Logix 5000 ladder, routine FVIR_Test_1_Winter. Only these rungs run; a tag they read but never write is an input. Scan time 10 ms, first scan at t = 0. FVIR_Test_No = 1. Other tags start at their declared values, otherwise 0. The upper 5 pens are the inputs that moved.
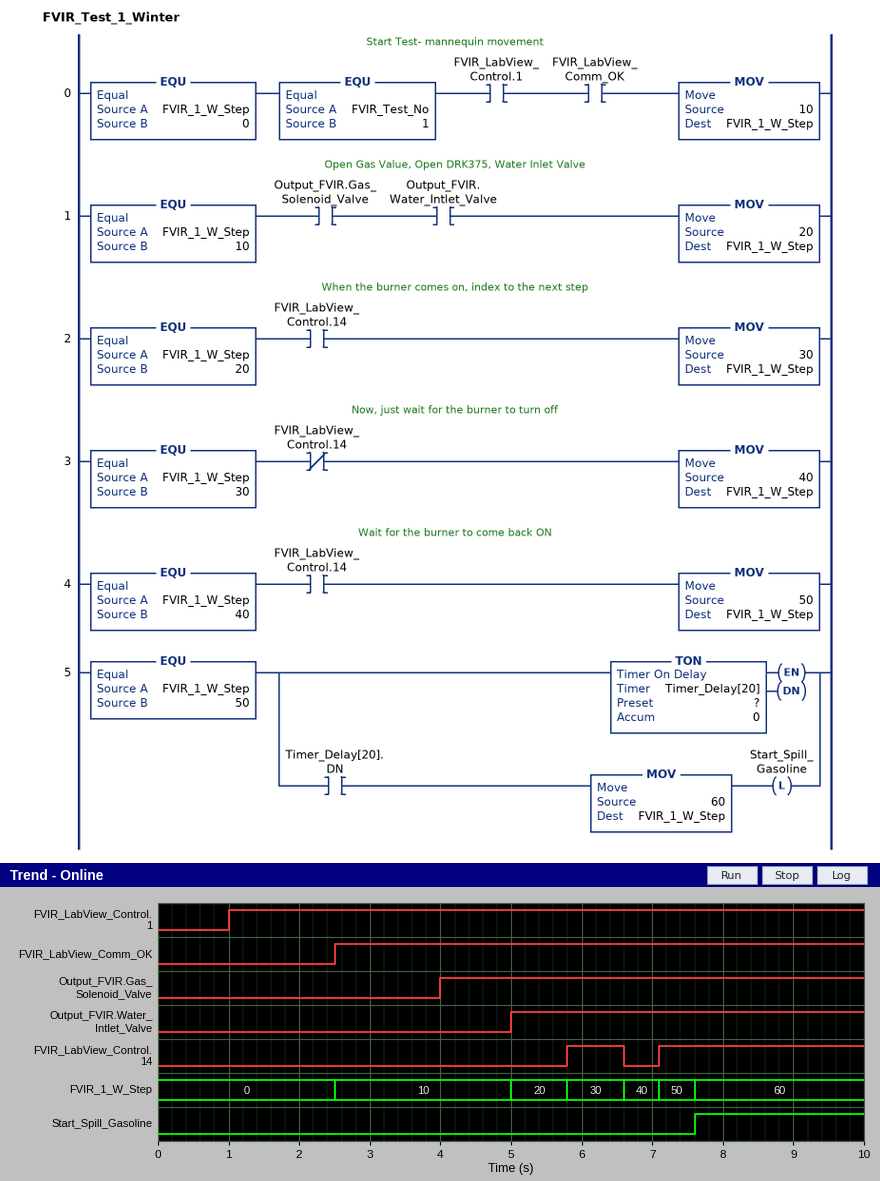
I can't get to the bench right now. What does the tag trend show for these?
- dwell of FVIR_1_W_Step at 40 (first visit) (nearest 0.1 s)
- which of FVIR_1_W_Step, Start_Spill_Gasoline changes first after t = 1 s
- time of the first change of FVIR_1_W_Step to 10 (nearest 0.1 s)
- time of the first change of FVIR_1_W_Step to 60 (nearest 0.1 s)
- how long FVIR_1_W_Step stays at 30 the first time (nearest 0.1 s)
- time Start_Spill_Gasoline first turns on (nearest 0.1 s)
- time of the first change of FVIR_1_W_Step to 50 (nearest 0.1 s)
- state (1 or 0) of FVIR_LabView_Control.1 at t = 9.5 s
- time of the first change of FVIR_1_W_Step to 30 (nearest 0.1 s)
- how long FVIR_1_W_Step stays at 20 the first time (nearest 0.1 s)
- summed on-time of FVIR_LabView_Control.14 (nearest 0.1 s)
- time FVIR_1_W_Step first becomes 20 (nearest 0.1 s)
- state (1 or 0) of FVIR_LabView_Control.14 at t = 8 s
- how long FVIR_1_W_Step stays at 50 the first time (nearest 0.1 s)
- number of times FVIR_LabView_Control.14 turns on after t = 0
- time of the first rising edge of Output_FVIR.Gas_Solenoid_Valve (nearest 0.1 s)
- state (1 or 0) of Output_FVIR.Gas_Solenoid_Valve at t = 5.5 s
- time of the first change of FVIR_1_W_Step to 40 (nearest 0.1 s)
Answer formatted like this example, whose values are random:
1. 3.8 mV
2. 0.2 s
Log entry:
1. 0.5 s
2. FVIR_1_W_Step
3. 2.5 s
4. 7.6 s
5. 0.8 s
6. 7.6 s
7. 7.1 s
8. 1
9. 5.8 s
10. 0.8 s
11. 3.7 s
12. 5.0 s
13. 1
14. 0.5 s
15. 2
16. 4.0 s
17. 1
18. 6.6 s
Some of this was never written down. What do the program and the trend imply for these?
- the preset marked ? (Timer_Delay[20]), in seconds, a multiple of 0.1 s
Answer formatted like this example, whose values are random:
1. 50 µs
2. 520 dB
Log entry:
1. 0.5 s
